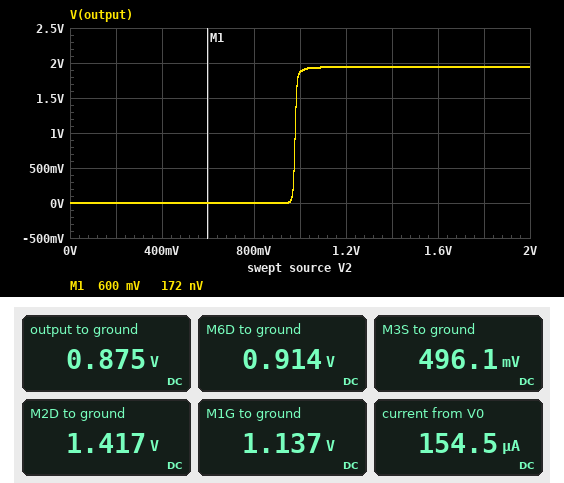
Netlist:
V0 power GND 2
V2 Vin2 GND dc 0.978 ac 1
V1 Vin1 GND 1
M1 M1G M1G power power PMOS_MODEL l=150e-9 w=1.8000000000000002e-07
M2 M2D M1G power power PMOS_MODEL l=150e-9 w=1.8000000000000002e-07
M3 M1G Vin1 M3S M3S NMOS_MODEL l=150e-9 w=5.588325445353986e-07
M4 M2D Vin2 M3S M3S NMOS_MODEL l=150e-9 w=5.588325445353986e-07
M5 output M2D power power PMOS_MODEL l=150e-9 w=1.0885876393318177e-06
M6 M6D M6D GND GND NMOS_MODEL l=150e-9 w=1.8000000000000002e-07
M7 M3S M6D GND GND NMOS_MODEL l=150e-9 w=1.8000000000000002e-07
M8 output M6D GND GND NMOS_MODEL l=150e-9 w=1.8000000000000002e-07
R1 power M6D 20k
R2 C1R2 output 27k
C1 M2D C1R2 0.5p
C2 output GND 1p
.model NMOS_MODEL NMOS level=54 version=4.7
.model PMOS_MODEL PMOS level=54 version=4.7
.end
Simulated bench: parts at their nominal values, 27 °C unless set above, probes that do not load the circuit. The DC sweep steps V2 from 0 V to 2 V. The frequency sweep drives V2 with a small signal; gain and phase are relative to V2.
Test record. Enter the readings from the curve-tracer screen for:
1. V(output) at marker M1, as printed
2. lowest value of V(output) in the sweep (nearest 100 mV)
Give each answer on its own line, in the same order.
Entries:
172 nV
0 V
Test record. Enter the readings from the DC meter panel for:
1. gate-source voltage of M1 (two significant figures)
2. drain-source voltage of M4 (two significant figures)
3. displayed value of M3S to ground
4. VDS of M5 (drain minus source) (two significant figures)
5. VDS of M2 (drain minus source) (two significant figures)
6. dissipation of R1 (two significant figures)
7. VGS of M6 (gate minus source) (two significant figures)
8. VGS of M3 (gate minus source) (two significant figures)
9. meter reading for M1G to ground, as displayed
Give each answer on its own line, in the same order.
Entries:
-860 mV
920 mV
496.1 mV
-1.1 V
-580 mV
59 µW
910 mV
500 mV
1.137 V
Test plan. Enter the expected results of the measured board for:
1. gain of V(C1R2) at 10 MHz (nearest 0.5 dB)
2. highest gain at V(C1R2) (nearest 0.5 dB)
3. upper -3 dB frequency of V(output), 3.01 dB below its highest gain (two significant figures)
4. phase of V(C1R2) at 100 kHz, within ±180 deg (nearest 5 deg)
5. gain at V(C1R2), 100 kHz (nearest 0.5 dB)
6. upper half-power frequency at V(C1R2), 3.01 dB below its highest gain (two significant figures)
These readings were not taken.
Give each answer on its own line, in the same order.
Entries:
16.0 dB
42.0 dB
440 kHz
-15 deg
41.5 dB
440 kHz
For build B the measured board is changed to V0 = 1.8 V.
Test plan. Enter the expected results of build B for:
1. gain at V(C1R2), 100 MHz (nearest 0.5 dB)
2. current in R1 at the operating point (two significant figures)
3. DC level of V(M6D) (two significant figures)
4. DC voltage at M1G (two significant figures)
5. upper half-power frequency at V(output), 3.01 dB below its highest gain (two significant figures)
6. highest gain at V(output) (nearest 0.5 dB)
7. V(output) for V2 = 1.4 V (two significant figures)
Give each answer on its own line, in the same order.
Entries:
11.0 dB
47 µA
860 mV
980 mV
420 kHz
41.5 dB
1.7 V
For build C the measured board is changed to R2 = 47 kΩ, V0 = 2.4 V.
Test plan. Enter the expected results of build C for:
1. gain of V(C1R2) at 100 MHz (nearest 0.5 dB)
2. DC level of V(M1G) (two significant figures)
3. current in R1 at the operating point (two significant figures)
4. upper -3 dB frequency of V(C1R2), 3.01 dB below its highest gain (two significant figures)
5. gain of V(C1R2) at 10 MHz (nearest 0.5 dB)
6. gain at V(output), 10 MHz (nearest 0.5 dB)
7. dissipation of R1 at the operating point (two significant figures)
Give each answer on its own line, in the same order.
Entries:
15.5 dB
1.5 V
69 µA
470 kHz
17.5 dB
20.0 dB
95 µW
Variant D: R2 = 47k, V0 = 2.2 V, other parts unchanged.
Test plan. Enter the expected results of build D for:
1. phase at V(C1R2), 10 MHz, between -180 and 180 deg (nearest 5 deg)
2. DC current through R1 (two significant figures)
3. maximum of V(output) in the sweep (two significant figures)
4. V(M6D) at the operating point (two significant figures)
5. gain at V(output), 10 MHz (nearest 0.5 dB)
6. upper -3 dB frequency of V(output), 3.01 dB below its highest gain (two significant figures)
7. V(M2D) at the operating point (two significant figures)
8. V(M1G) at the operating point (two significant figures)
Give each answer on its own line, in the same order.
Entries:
-110 deg
62 µA
2.1 V
970 mV
19.5 dB
450 kHz
1.6 V
1.3 V
